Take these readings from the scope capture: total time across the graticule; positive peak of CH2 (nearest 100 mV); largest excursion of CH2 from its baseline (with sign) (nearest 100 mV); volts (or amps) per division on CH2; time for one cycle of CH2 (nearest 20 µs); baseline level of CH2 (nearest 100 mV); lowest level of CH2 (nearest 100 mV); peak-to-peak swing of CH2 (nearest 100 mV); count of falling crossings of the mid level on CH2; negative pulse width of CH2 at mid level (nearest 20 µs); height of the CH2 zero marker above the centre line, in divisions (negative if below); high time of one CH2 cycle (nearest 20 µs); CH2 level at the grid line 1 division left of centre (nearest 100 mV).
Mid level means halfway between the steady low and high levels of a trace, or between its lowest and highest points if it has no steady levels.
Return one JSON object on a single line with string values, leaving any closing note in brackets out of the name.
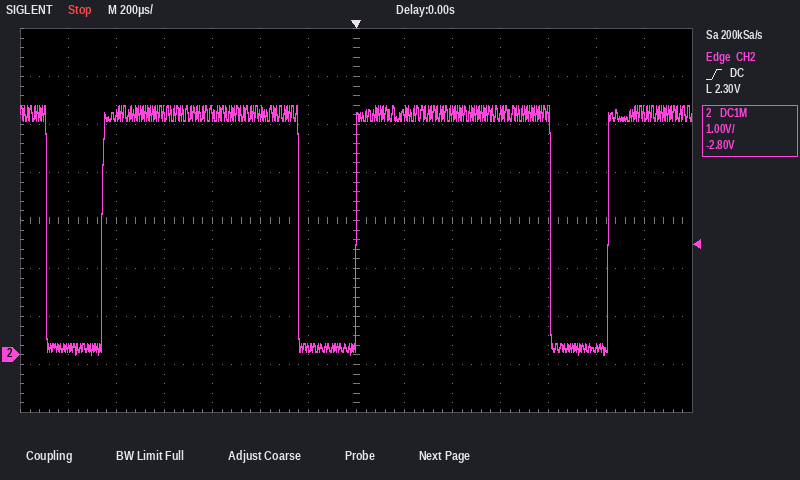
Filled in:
{"total time across the graticule": "2.8 ms", "positive peak of CH2": "5.2 V", "largest excursion of CH2 from its baseline (with sign)": "-5.0 V", "volts (or amps) per division on CH2": "1 V", "time for one cycle of CH2": "1.06 ms", "baseline level of CH2": "5.0 V", "lowest level of CH2": "0.0 V", "peak-to-peak swing of CH2": "5.2 V", "count of falling crossings of the mid level on CH2": "3", "negative pulse width of CH2 at mid level": "240 µs", "height of the CH2 zero marker above the centre line, in divisions": "-2.8 div", "high time of one CH2 cycle": "820 µs", "CH2 level at the grid line 1 division left of centre": "200 mV"}
